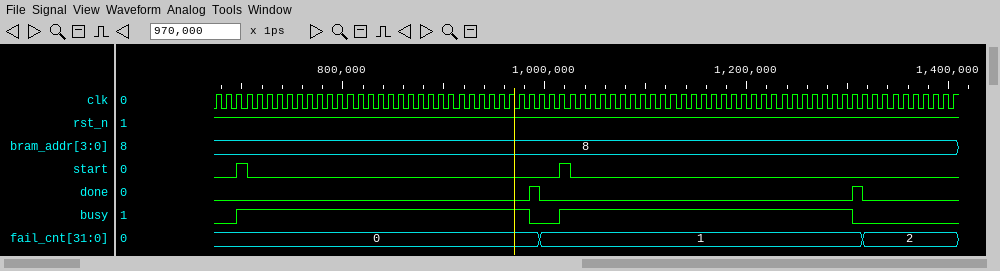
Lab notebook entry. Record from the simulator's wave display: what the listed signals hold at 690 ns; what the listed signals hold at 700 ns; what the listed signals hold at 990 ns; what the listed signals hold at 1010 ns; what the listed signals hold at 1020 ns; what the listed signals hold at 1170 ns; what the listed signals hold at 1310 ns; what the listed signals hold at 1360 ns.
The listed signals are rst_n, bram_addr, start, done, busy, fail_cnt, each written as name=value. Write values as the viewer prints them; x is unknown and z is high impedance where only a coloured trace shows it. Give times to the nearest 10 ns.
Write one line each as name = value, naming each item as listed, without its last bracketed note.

what the listed signals hold at 690 ns = rst_n=1, bram_addr=8, start=0, done=0, busy=0, fail_cnt=0
what the listed signals hold at 700 ns = rst_n=1, bram_addr=8, start=1, done=0, busy=1, fail_cnt=0
what the listed signals hold at 990 ns = rst_n=1, bram_addr=8, start=0, done=1, busy=0, fail_cnt=0
what the listed signals hold at 1010 ns = rst_n=1, bram_addr=8, start=0, done=0, busy=0, fail_cnt=1
what the listed signals hold at 1020 ns = rst_n=1, bram_addr=8, start=1, done=0, busy=1, fail_cnt=1
what the listed signals hold at 1170 ns = rst_n=1, bram_addr=8, start=0, done=0, busy=1, fail_cnt=1
what the listed signals hold at 1310 ns = rst_n=1, bram_addr=8, start=0, done=1, busy=0, fail_cnt=1
what the listed signals hold at 1360 ns = rst_n=1, bram_addr=8, start=0, done=0, busy=0, fail_cnt=2
